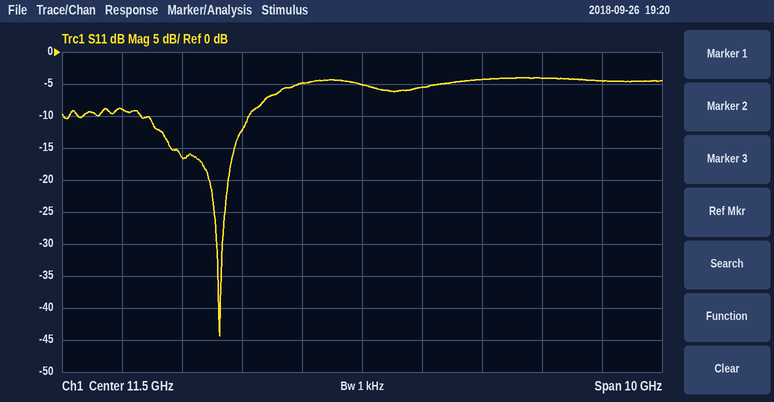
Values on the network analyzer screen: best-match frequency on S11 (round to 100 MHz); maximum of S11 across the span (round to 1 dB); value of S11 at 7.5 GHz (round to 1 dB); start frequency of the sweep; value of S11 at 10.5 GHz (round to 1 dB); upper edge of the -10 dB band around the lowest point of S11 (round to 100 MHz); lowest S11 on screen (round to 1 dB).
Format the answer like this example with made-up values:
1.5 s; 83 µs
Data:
9.1 GHz; -4 dB; -9 dB; 6.5 GHz; -5 dB; 9.6 GHz; -44 dB
